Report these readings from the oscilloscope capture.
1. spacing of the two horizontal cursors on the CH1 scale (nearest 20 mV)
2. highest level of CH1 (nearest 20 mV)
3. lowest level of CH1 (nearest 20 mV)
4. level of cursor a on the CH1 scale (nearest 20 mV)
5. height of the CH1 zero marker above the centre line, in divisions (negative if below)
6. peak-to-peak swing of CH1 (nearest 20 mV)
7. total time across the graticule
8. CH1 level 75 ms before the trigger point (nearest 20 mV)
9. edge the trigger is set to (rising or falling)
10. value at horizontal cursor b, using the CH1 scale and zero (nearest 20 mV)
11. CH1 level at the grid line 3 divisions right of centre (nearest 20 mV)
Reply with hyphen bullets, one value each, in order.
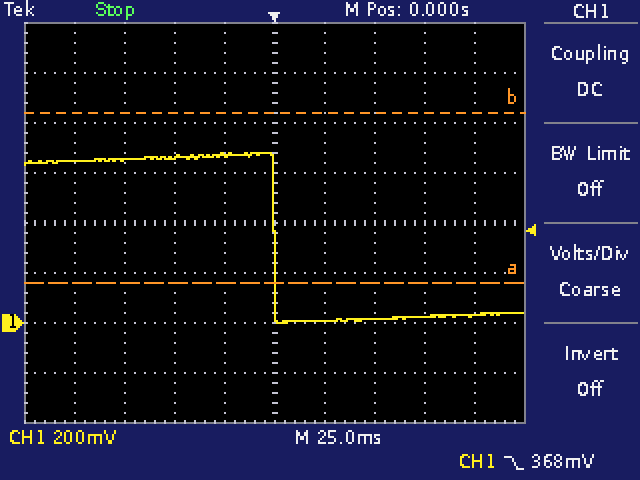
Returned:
- 680 mV
- 680 mV
- 0 mV
- 160 mV
- -2.0 div
- 680 mV
- 250 ms
- 660 mV
- falling
- 840 mV
- 20 mV
